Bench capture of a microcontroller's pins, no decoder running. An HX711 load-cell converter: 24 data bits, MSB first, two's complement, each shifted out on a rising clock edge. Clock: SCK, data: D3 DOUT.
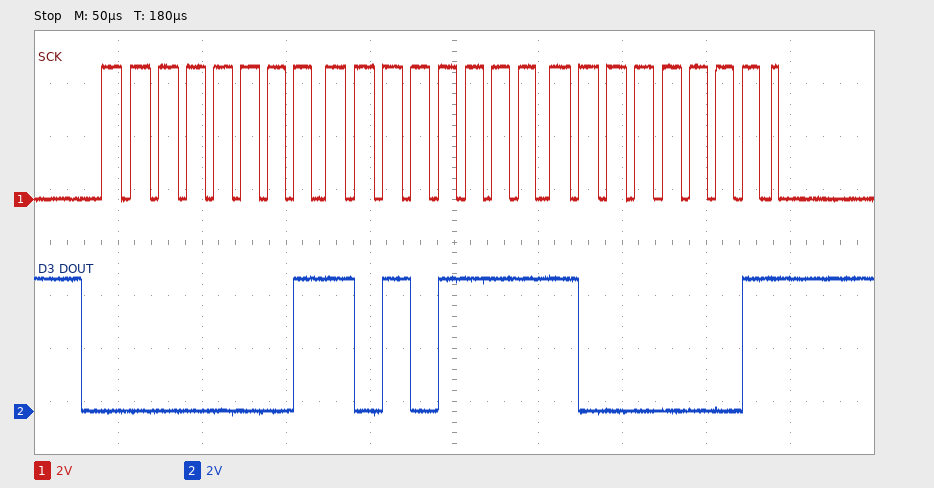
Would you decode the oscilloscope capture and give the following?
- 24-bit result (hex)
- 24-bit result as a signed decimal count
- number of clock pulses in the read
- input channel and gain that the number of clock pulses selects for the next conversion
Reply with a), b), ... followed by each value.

a) 0x01AF81
b) 110465
c) 25
d) channel A, gain 128
